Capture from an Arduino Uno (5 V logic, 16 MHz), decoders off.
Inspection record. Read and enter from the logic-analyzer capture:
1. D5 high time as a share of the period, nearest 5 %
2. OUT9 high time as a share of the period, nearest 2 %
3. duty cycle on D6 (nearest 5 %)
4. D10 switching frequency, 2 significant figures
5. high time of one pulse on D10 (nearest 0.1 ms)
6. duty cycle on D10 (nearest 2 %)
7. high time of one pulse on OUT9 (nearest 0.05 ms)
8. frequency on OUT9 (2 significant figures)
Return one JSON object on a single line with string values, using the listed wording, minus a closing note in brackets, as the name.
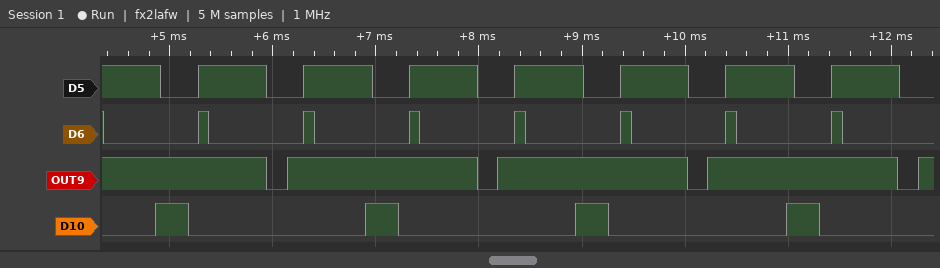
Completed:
{"D5 high time as a share of the period, nearest 5 %": "65 %", "OUT9 high time as a share of the period, nearest 2 %": "90 %", "duty cycle on D6": "10 %", "D10 switching frequency, 2 significant figures": "490 Hz", "high time of one pulse on D10": "0.3 ms", "duty cycle on D10": "16 %", "high time of one pulse on OUT9": "1.85 ms", "frequency on OUT9": "490 Hz"}
